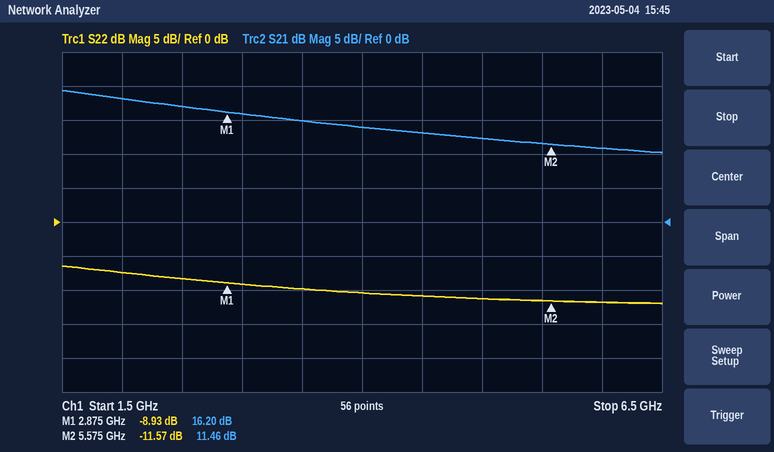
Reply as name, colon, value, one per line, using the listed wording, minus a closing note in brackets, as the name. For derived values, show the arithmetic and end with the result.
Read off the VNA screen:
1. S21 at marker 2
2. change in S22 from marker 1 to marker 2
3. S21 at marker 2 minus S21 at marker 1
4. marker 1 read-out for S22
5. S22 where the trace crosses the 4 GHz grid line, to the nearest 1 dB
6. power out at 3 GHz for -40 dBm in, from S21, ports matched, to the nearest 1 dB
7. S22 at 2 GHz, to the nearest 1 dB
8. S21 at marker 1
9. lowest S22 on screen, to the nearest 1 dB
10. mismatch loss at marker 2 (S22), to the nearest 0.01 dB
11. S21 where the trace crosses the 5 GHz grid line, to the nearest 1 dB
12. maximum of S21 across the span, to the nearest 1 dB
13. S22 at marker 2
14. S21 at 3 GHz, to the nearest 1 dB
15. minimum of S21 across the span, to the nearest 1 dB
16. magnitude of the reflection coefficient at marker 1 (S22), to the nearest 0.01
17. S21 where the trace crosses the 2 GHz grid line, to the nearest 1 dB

S21 at marker 2: 11.46 dB
change in S22 from marker 1 to marker 2: -11.57 − (-8.93) = -2.64 dB
S21 at marker 2 minus S21 at marker 1: 11.46 − (16.2) = -4.74 dB
marker 1 read-out for S22: -8.93 dB
S22 where the trace crosses the 4 GHz grid line, to the nearest 1 dB: -10 dB
power out at 3 GHz for -40 dBm in, from S21, ports matched, to the nearest 1 dB: -40 dBm + (16 dB) = -24 dBm
S22 at 2 GHz, to the nearest 1 dB: -7 dB
S21 at marker 1: 16.20 dB
lowest S22 on screen, to the nearest 1 dB: -12 dB
mismatch loss at marker 2 (S22), to the nearest 0.01 dB: −10 log10(1 − 10^(-11.57/10)) ≈ 0.31 dB
S21 where the trace crosses the 5 GHz grid line, to the nearest 1 dB: 12 dB
maximum of S21 across the span, to the nearest 1 dB: 19 dB
S22 at marker 2: -11.57 dB
S21 at 3 GHz, to the nearest 1 dB: 16 dB
minimum of S21 across the span, to the nearest 1 dB: 10 dB
magnitude of the reflection coefficient at marker 1 (S22), to the nearest 0.01: 10^(-8.93/20) ≈ 0.36
S21 where the trace crosses the 2 GHz grid line, to the nearest 1 dB: 18 dB
